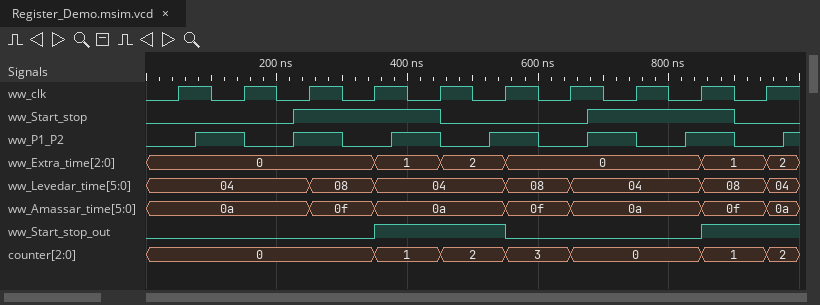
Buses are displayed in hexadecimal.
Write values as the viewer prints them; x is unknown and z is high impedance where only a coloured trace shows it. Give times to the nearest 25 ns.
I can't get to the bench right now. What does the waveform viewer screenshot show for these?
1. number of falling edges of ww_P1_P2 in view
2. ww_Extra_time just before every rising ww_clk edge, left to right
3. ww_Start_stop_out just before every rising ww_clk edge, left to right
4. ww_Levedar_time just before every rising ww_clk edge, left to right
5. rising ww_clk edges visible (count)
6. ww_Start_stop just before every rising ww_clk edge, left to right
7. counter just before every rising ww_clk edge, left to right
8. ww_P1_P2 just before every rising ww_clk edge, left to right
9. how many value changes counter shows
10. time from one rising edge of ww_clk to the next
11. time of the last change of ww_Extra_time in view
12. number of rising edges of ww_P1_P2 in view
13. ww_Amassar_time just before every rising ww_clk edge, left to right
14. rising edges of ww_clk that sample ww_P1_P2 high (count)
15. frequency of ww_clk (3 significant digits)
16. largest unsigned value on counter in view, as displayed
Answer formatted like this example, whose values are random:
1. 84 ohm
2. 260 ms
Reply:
1. 6
2. 0, 0, 0, 0, 1, 2, 0, 0, 0, 1
3. 0 0 0 0 1 1 0 0 0 1
4. 04, 04, 04, 08, 04, 04, 08, 04, 04, 08
5. 10
6. 0 0 1 1 1 0 0 1 1 0
7. 0, 0, 0, 0, 1, 2, 3, 0, 0, 1
8. 0 1 1 0 1 1 0 1 1 0
9. 6
10. 100 ns
11. 950 ns
12. 7
13. 0a, 0a, 0a, 0f, 0a, 0a, 0f, 0a, 0a, 0f
14. 6
15. 10.0 MHz
16. 3
